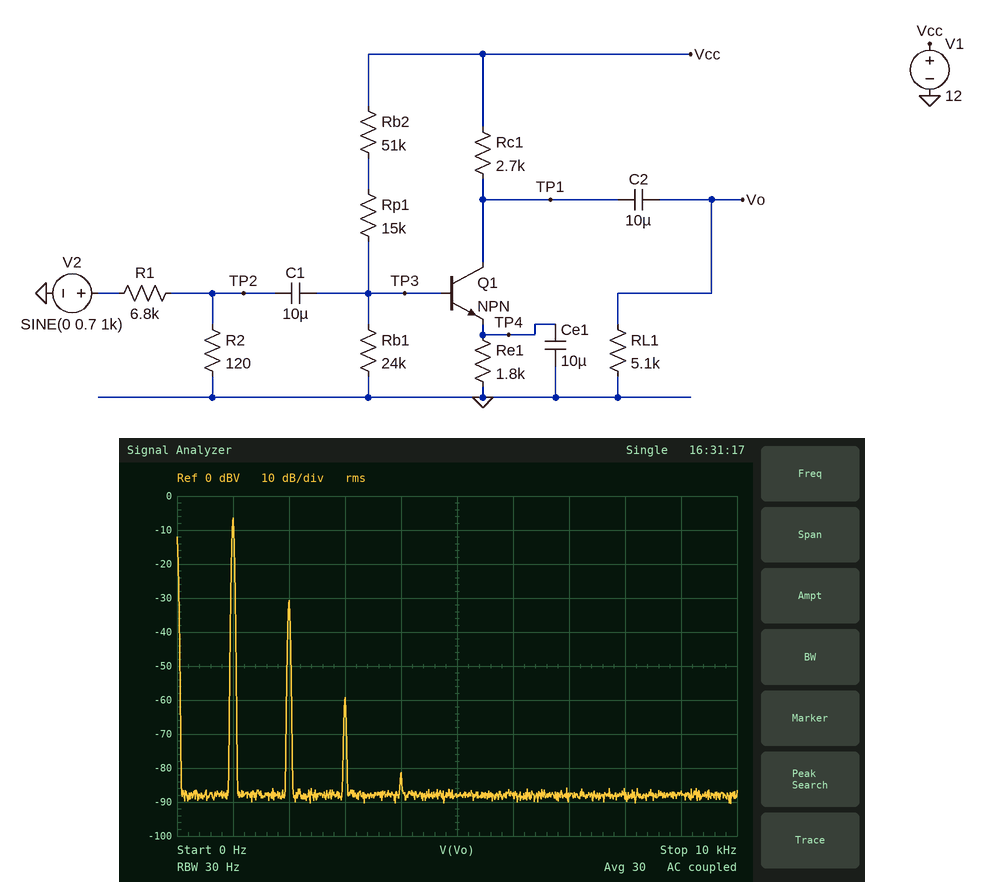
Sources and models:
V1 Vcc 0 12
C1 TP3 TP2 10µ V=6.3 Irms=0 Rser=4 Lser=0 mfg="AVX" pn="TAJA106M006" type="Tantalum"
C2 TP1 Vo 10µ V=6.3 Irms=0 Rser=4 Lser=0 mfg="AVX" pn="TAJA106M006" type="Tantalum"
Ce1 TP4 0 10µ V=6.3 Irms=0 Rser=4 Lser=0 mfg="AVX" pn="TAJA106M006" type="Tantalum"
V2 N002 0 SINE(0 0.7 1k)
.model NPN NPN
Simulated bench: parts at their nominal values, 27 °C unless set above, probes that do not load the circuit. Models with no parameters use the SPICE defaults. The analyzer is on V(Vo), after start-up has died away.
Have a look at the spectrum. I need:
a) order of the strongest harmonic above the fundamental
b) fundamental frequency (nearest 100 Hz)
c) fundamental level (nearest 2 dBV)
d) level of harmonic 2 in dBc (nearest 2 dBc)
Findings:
2
1.0 kHz
-6 dBV
-24 dBc
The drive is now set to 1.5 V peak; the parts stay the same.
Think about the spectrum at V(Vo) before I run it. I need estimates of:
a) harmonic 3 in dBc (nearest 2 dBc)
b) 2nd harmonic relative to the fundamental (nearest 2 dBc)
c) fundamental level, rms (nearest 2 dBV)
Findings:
-40 dBc
-18 dBc
0 dBV
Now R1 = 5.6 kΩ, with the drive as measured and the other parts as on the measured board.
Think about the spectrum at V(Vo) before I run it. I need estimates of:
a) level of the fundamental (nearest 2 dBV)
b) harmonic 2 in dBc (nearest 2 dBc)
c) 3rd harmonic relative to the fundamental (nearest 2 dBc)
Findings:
-4 dBV
-22 dBc
-50 dBc
